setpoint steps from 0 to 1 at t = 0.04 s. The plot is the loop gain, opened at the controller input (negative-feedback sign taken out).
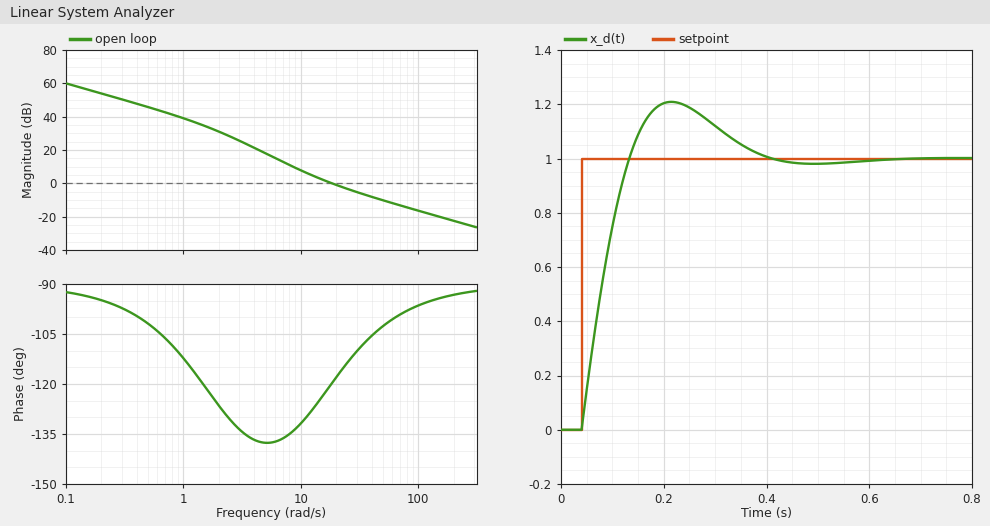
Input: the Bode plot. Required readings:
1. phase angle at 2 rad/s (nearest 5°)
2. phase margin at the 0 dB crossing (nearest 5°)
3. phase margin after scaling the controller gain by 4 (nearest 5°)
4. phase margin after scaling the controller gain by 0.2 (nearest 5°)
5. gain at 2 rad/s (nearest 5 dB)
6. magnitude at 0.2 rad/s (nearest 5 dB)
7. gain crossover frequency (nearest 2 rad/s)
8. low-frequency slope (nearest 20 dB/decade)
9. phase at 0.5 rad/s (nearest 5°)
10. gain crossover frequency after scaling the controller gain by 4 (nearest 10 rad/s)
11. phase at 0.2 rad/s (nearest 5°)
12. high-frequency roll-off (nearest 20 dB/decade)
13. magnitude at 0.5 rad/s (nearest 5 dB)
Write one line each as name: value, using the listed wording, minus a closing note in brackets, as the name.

phase angle at 2 rad/s: -125°
phase margin at the 0 dB crossing: 60°
phase margin after scaling the controller gain by 4: 80°
phase margin after scaling the controller gain by 0.2: 45°
gain at 2 rad/s: 30 dB
magnitude at 0.2 rad/s: 55 dB
gain crossover frequency: 18 rad/s
low-frequency slope: -20 dB/decade
phase at 0.5 rad/s: -100°
gain crossover frequency after scaling the controller gain by 4: 60 rad/s
phase at 0.2 rad/s: -95°
high-frequency roll-off: -20 dB/decade
magnitude at 0.5 rad/s: 45 dB
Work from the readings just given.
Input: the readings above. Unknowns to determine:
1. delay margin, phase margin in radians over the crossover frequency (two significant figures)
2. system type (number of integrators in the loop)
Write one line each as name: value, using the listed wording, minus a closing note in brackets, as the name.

delay margin, phase margin in radians over the crossover frequency: 0.058 s
system type: 1
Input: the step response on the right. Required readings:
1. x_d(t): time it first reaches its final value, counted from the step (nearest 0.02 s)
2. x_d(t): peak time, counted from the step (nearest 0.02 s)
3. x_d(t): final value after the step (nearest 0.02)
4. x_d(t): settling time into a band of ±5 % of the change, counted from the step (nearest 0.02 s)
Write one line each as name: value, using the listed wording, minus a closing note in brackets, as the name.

x_d(t): time it first reaches its final value, counted from the step: 0.10 s
x_d(t): peak time, counted from the step: 0.18 s
x_d(t): final value after the step: 1.00
x_d(t): settling time into a band of ±5 % of the change, counted from the step: 0.32 s
